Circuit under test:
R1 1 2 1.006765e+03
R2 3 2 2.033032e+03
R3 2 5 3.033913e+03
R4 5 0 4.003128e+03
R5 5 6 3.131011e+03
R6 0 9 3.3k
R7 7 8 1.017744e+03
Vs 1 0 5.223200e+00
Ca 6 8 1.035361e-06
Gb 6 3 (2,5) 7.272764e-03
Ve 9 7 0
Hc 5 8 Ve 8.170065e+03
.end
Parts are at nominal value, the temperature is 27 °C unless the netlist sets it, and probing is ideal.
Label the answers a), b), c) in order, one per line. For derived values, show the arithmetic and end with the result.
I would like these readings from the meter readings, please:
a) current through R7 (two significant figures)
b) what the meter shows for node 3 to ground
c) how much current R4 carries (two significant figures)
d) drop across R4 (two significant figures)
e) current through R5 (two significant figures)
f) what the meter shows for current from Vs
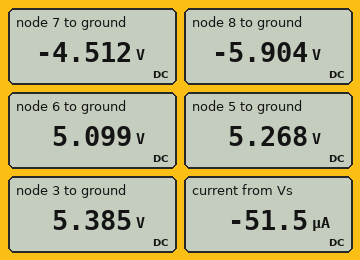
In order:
a) (-4.512 V - (-5.904 V)) / 1.018 kΩ = 1.4 mA
b) 5.385 V
c) (5.268 V) / 4.003 kΩ = 1.3 mA
d) 5.268 V = 5.3 V
e) (5.268 V - 5.099 V) / 3.131 kΩ = 54 µA
f) -51.5 µA
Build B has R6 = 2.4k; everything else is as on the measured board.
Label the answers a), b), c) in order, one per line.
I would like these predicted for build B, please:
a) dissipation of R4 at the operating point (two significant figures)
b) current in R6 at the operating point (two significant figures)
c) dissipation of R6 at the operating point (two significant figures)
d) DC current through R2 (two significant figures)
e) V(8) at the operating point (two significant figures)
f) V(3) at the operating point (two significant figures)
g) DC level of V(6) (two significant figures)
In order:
a) 6.4 mW
b) 1.1 mA
c) 2.7 mW
d) 210 µA
e) -3.6 V
f) 4.6 V
g) 5.7 V
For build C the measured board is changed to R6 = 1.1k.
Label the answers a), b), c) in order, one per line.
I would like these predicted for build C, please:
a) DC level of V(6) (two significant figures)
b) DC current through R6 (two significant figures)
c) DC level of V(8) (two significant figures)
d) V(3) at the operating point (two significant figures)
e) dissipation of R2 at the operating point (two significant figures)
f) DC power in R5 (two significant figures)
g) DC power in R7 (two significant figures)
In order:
a) 6.2 V
b) 800 µA
c) -1.7 V
d) 3.9 V
e) 380 µW
f) 580 µW
g) 660 µW
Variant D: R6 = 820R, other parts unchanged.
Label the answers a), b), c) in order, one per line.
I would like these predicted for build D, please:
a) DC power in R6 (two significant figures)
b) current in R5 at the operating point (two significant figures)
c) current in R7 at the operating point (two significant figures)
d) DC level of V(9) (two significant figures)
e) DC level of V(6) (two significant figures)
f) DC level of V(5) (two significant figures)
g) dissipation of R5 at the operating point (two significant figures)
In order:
a) 480 µW
b) 470 µA
c) 760 µA
d) -630 mV
e) 6.3 V
f) 4.8 V
g) 680 µW
